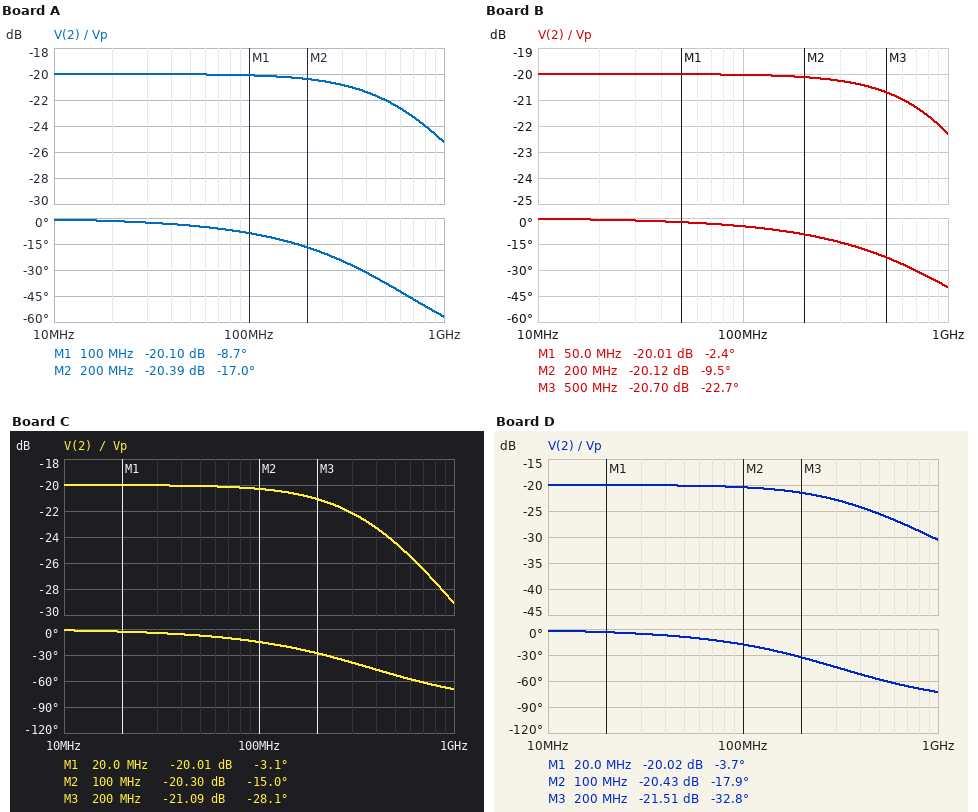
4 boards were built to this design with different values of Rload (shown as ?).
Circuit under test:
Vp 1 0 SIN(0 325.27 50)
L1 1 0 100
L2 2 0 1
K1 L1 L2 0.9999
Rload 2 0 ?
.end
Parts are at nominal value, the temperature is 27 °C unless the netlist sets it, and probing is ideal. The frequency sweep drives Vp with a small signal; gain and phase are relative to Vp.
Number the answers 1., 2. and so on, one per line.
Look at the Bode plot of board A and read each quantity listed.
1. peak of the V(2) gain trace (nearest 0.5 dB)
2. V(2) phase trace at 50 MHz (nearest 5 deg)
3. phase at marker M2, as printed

1. -20.0 dB
2. -5 deg
3. -17.0 deg
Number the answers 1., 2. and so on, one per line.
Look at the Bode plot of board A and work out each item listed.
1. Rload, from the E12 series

1. 820 kΩ
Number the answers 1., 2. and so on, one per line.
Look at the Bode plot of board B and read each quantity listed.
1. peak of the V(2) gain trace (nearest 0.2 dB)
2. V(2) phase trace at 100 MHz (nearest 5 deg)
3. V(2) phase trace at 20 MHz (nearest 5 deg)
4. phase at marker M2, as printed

1. -20.0 dB
2. -5 deg
3. 0 deg
4. -9.5 deg
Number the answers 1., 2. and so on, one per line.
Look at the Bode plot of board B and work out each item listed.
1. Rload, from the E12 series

1. 1.5 MΩ
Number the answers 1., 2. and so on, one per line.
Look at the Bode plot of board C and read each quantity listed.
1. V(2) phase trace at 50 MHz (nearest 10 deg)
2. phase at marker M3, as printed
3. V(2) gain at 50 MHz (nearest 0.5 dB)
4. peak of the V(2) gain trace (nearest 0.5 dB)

1. -10 deg
2. -28.1 deg
3. -20.0 dB
4. -20.0 dB
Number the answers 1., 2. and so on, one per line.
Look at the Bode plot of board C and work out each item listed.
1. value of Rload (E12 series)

1. 470 kΩ
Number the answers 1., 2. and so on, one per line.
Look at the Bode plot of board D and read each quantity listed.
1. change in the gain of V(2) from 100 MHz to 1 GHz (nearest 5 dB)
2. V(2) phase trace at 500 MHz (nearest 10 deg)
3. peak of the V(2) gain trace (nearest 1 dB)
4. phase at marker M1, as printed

1. -10 dB
2. -60 deg
3. -20 dB
4. -3.7 deg
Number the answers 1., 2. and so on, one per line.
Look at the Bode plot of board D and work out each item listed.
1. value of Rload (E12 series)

1. 390 kΩ
